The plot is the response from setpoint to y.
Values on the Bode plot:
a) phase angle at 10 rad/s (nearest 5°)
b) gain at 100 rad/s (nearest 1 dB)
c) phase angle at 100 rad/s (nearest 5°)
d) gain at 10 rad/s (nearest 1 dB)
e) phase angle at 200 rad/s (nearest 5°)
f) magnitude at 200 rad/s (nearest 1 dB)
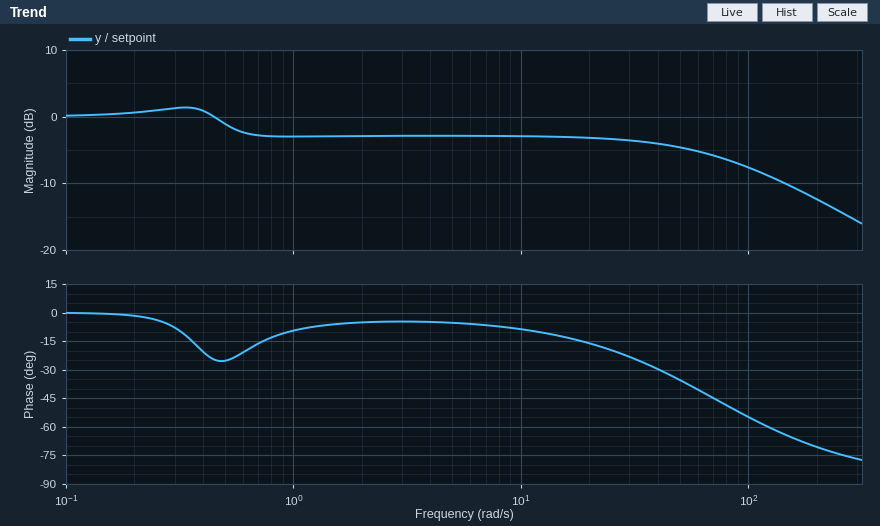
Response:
-10°
-8 dB
-55°
-3 dB
-70°
-12 dB
